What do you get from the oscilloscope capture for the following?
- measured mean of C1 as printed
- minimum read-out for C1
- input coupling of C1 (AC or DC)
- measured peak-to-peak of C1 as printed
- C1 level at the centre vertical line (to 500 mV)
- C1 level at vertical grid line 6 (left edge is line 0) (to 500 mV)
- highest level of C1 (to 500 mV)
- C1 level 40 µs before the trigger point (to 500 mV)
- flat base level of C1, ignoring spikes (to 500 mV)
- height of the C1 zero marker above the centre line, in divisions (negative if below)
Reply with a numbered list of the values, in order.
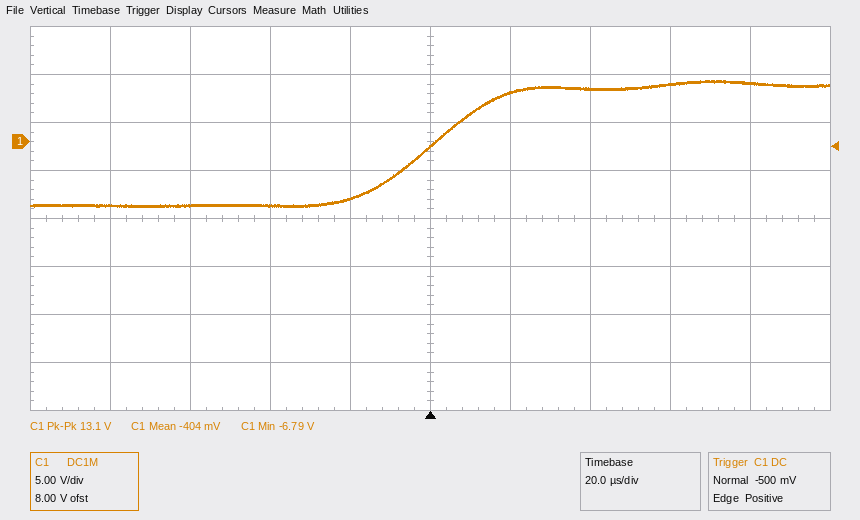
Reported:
1. -404 mV
2. -6.79 V
3. DC
4. 13.1 V
5. -500 mV
6. 5.0 V
7. 6.5 V
8. -6.5 V
9. -6.5 V
10. +1.6 div
